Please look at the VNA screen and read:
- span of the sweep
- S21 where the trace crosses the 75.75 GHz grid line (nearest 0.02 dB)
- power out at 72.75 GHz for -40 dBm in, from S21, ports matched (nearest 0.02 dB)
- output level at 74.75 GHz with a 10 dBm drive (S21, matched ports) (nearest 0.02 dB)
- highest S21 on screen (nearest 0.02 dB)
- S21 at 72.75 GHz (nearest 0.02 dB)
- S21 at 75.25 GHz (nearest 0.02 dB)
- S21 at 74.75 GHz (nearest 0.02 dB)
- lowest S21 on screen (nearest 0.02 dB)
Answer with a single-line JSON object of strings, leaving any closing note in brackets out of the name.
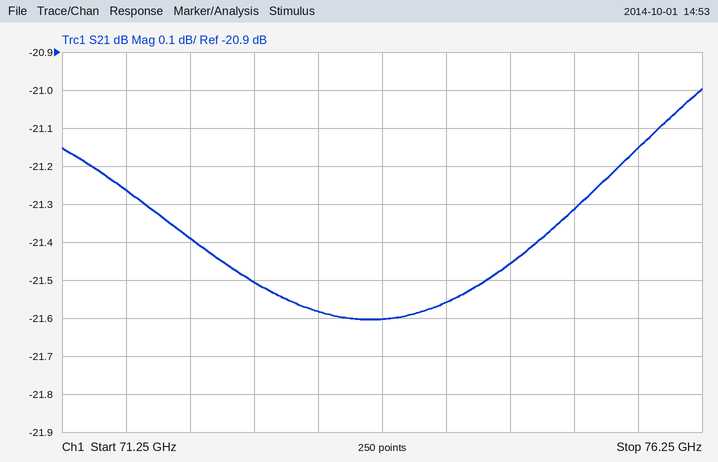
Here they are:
{"span of the sweep": "5 GHz", "S21 where the trace crosses the 75.75 GHz grid line": "-21.16 dB", "power out at 72.75 GHz for -40 dBm in, from S21, ports matched": "-61.50 dBm", "output level at 74.75 GHz with a 10 dBm drive (S21, matched ports)": "-11.46 dBm", "highest S21 on screen": "-21.00 dB", "S21 at 72.75 GHz": "-21.50 dB", "S21 at 75.25 GHz": "-21.32 dB", "S21 at 74.75 GHz": "-21.46 dB", "lowest S21 on screen": "-21.60 dB"}
